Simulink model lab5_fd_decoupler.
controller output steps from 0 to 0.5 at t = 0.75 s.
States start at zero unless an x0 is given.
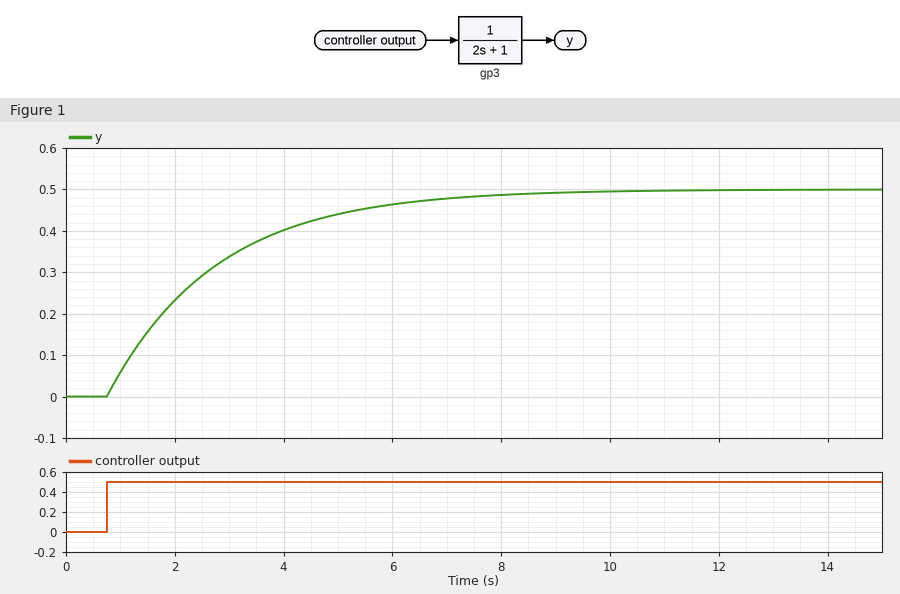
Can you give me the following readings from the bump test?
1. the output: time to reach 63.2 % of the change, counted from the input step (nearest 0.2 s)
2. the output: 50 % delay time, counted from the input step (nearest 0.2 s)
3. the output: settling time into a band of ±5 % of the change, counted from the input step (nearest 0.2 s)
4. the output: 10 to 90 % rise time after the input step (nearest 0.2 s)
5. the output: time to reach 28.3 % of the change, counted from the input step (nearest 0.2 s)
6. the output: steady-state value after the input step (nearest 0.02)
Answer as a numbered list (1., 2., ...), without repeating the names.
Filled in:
1. 2.0 s
2. 1.4 s
3. 6.0 s
4. 4.4 s
5. 0.6 s
6. 0.50
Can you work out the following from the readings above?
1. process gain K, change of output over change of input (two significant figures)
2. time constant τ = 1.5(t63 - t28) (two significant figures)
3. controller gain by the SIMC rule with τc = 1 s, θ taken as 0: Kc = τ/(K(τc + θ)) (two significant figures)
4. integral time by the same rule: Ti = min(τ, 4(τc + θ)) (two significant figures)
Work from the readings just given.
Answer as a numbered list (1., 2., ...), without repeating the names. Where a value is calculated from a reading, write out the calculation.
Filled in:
1. (0.5 - 0) / 0.5 = 1.0
2. 1.5 × (2 - 0.6) = 2.1 s
3. 2.1 / (1 × (1 + 0)) = 2.1
4. min(2.1, 4 × (1 + 0)) = 2.1 s
